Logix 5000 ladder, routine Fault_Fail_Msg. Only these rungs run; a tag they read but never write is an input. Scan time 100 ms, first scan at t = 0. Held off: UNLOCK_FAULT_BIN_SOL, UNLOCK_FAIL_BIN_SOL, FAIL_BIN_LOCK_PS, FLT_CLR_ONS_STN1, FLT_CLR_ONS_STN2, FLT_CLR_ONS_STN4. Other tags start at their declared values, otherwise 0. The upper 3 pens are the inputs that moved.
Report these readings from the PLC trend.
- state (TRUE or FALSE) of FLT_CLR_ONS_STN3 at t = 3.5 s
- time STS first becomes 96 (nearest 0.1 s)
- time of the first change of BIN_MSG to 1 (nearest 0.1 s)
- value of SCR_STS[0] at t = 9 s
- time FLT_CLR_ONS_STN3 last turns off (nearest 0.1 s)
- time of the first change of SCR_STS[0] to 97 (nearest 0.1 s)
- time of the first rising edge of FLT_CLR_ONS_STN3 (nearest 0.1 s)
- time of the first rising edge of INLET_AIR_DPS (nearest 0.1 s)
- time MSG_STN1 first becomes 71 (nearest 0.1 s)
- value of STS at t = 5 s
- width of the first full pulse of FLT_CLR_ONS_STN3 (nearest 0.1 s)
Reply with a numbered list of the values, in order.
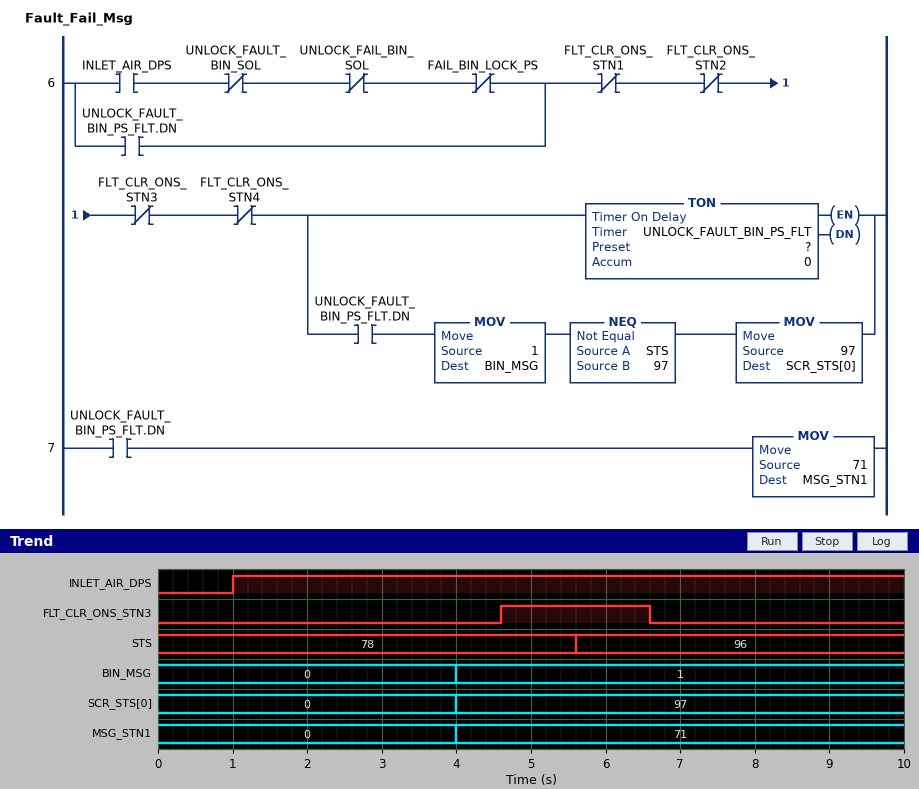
1. FALSE
2. 5.6 s
3. 4.0 s
4. 97
5. 6.6 s
6. 4.0 s
7. 4.6 s
8. 1.0 s
9. 4.0 s
10. 78
11. 2.0 s
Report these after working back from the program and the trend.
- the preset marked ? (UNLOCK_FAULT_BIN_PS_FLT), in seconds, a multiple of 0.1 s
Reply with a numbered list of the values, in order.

1. 3.0 s
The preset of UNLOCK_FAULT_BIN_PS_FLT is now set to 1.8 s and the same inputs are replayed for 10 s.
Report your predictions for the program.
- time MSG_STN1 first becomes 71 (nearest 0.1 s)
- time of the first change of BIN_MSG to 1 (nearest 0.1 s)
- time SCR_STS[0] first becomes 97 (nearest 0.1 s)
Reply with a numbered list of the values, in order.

1. 2.8 s
2. 2.8 s
3. 2.8 s
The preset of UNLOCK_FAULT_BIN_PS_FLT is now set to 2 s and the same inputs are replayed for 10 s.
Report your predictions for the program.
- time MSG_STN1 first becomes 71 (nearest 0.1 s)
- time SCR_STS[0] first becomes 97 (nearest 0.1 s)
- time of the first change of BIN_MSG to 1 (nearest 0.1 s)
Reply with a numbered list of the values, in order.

1. 3.0 s
2. 3.0 s
3. 3.0 s
